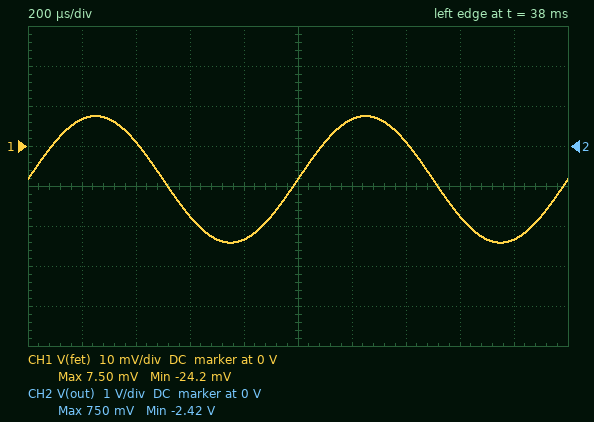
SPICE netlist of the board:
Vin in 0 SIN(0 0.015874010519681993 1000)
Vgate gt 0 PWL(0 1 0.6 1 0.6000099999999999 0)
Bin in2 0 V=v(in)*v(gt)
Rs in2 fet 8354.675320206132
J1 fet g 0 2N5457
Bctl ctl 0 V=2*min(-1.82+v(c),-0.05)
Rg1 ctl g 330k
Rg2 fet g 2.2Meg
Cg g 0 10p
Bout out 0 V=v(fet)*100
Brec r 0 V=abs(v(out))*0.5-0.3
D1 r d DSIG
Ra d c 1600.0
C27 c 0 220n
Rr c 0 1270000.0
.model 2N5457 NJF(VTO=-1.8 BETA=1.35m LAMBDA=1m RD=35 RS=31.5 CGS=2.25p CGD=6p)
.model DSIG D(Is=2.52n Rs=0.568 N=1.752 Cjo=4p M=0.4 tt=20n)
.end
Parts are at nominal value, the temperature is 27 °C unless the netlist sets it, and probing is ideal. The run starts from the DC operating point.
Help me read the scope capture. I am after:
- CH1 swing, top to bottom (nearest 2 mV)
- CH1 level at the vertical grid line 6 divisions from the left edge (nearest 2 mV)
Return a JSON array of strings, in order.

["32 mV", "6 mV"]
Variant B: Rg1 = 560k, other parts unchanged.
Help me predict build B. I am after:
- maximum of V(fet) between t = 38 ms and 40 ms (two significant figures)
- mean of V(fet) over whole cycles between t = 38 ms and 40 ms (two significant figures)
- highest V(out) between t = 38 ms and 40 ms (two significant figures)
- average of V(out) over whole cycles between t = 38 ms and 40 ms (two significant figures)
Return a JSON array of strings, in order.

["8.0 mV", "-7.8 mV", "800 mV", "-780 mV"]
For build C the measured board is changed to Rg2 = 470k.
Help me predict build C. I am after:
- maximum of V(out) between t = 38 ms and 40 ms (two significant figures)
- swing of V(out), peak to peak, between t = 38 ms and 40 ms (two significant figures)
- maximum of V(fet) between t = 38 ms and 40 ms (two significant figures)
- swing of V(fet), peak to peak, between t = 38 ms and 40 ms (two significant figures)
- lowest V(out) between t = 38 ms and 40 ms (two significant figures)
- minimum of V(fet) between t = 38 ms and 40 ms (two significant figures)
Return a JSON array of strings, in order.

["-610 mV", "1.3 V", "-6.1 mV", "13 mV", "-1.9 V", "-19 mV"]
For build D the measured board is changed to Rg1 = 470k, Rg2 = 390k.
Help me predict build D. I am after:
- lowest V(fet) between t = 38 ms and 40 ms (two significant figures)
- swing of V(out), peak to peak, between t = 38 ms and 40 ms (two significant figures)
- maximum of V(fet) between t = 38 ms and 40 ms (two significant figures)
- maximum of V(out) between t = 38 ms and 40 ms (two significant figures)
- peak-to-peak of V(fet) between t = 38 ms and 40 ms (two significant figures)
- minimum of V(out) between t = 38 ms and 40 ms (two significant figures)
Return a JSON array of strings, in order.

["-11 mV", "670 mV", "-4.0 mV", "-400 mV", "6.7 mV", "-1.1 V"]
